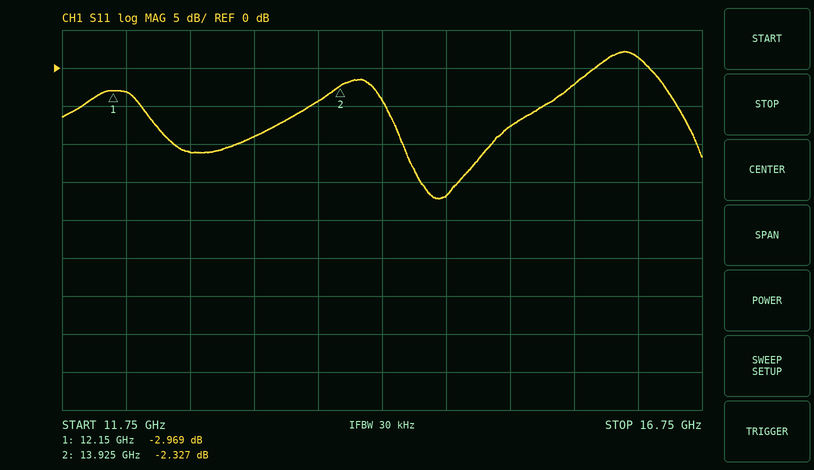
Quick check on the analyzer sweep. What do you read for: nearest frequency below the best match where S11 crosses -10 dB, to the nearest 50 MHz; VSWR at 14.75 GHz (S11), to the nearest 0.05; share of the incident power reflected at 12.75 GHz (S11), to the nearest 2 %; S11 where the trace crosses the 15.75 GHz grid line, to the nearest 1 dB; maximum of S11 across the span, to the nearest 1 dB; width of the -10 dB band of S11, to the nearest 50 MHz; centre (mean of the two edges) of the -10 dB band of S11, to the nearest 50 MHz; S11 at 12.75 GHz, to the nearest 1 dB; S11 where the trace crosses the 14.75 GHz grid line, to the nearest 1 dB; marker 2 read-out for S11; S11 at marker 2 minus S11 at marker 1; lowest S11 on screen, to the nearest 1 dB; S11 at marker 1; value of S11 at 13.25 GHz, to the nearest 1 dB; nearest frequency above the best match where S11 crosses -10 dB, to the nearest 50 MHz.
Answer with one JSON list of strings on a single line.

["14.40 GHz", "1.35", "8 %", "-2 dB", "2 dB", "700 MHz", "14.75 GHz", "-11 dB", "-17 dB", "-2.327 dB", "0.642 dB", "-17 dB", "-2.969 dB", "-9 dB", "15.10 GHz"]
